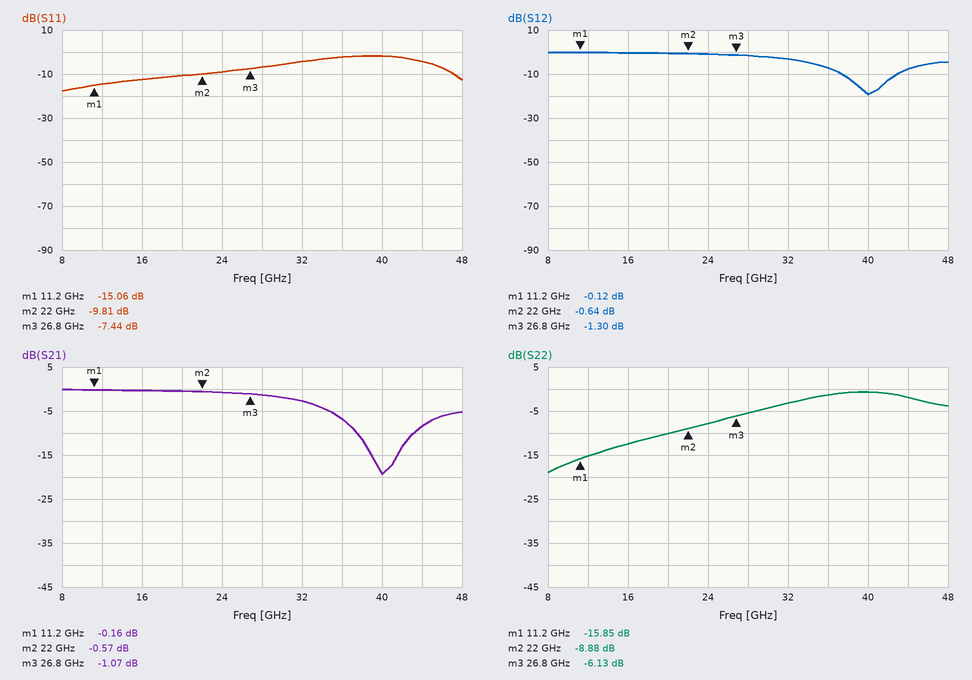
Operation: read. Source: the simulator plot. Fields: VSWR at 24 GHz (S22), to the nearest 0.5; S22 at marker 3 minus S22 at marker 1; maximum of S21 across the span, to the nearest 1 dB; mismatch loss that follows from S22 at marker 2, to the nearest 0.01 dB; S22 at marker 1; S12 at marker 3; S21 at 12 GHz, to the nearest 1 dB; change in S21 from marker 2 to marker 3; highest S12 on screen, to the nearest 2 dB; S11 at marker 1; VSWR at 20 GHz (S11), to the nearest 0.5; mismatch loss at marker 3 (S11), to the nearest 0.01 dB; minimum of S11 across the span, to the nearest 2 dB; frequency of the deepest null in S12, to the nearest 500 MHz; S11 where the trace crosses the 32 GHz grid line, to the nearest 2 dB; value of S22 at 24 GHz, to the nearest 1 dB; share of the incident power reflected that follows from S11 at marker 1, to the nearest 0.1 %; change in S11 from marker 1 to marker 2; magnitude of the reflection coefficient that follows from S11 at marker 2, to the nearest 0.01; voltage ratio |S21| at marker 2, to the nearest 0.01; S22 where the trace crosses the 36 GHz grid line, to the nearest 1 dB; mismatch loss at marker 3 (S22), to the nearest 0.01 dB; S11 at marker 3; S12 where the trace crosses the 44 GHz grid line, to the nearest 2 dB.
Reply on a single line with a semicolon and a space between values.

2.5; 9.72 dB; 0 dB; 0.60 dB; -15.85 dB; -1.30 dB; 0 dB; -0.50 dB; 0 dB; -15.06 dB; 2.0; 0.86 dB; -18 dB; 40.0 GHz; -4 dB; -8 dB; 3.1 %; 5.25 dB; 0.32; 0.94; -1 dB; 1.21 dB; -7.44 dB; -8 dB
